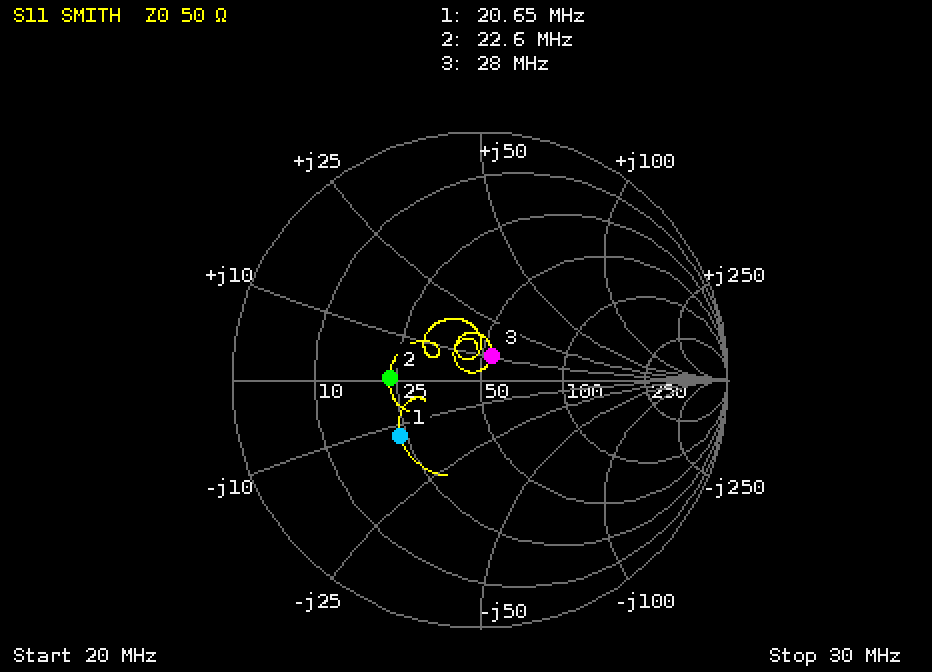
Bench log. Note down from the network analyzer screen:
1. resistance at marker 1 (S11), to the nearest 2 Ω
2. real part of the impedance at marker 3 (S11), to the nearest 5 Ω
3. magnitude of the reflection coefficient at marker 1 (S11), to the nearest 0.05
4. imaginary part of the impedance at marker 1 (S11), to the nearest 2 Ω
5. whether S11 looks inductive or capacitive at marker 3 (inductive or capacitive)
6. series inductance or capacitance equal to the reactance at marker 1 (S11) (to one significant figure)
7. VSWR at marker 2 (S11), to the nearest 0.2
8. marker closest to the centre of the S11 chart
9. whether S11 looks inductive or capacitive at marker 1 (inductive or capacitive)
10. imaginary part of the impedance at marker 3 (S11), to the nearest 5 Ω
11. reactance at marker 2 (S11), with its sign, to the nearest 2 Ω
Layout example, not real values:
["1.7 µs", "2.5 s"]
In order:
["24 Ω", "55 Ω", "0.40", "-12 Ω", "inductive", "600 pF", "2.2", "marker 3", "capacitive", "+10 Ω", "0 Ω"]
